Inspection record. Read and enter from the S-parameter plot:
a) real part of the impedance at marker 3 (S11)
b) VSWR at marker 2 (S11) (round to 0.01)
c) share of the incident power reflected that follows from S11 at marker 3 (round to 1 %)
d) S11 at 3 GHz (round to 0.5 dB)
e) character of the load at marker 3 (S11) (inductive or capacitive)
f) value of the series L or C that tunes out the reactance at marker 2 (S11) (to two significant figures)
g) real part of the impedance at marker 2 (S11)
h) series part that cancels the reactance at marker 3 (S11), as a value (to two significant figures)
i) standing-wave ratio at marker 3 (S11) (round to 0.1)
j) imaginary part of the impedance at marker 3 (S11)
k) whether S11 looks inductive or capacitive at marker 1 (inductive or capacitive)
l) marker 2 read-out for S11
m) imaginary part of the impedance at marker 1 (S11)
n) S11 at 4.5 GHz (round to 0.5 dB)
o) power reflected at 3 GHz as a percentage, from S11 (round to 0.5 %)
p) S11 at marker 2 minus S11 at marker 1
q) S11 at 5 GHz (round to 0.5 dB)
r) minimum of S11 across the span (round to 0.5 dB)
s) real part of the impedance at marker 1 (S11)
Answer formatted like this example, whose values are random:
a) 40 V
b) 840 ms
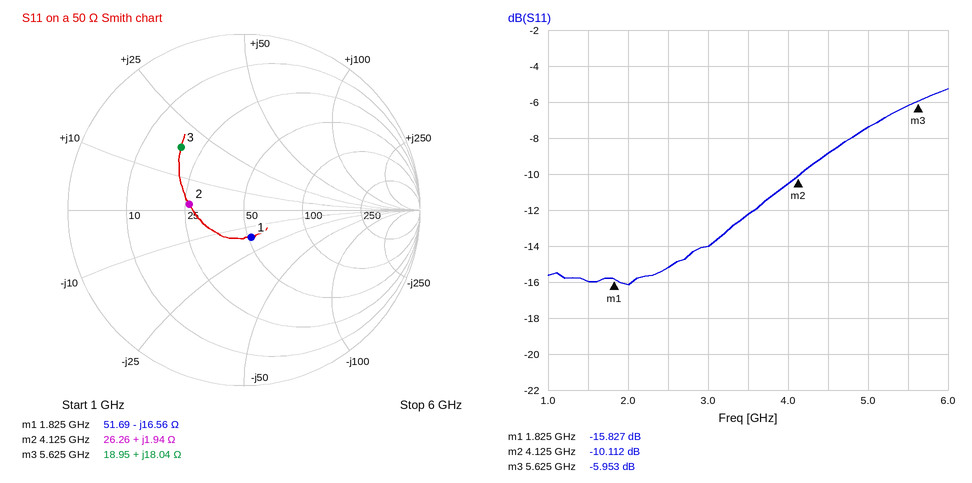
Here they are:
a) 18.95 Ω
b) 1.91
c) 25 %
d) -14.0 dB
e) inductive
f) 20 pF
g) 26.26 Ω
h) 1.6 pF
i) 3.0
j) +18.04 Ω
k) capacitive
l) -10.112 dB
m) -16.56 Ω
n) -9.0 dB
o) 4.0 %
p) 5.715 dB
q) -7.5 dB
r) -16.0 dB
s) 51.69 Ω
